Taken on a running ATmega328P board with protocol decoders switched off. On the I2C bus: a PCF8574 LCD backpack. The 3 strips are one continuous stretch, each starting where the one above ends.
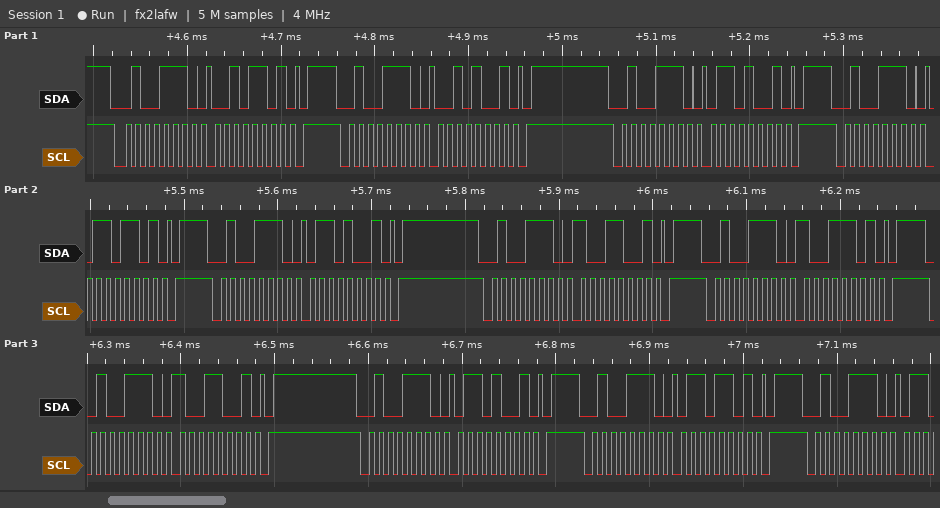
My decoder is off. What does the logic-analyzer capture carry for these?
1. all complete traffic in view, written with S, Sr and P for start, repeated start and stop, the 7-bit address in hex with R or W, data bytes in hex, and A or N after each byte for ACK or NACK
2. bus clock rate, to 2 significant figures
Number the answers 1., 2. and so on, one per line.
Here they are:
1. S 27W A 2D A P S 27W A 29 A P S 27W A 69 A P S 27W A 6D A P S 27W A 69 A P S 27W A 99 A P S 27W A 9D A P S 27W A 99 A P S 27W A 69 A P S 27W A 6D A P S 27W A
2. 100 kHz
